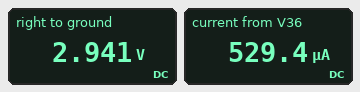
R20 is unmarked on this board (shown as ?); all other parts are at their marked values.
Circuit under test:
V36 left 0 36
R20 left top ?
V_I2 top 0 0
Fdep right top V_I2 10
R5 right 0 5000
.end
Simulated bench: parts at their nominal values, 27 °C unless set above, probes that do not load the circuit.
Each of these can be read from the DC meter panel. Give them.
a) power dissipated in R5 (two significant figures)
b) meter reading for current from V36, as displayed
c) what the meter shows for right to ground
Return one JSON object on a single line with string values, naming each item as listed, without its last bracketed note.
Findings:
{"power dissipated in R5": "1.7 mW", "meter reading for current from V36, as displayed": "529.4 µA", "what the meter shows for right to ground": "2.941 V"}
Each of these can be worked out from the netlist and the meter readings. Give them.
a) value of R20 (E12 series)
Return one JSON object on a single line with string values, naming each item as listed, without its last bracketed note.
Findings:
{"value of R20": "68 kΩ"}
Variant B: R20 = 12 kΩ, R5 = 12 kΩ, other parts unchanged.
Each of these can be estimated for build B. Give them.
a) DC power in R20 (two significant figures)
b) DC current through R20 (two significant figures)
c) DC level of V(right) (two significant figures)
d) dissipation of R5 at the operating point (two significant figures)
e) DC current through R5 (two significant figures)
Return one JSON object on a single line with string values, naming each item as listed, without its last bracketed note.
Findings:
{"DC power in R20": "110 mW", "DC current through R20": "3.0 mA", "DC level of V(right)": "40 V", "dissipation of R5 at the operating point": "130 mW", "DC current through R5": "3.3 mA"}
